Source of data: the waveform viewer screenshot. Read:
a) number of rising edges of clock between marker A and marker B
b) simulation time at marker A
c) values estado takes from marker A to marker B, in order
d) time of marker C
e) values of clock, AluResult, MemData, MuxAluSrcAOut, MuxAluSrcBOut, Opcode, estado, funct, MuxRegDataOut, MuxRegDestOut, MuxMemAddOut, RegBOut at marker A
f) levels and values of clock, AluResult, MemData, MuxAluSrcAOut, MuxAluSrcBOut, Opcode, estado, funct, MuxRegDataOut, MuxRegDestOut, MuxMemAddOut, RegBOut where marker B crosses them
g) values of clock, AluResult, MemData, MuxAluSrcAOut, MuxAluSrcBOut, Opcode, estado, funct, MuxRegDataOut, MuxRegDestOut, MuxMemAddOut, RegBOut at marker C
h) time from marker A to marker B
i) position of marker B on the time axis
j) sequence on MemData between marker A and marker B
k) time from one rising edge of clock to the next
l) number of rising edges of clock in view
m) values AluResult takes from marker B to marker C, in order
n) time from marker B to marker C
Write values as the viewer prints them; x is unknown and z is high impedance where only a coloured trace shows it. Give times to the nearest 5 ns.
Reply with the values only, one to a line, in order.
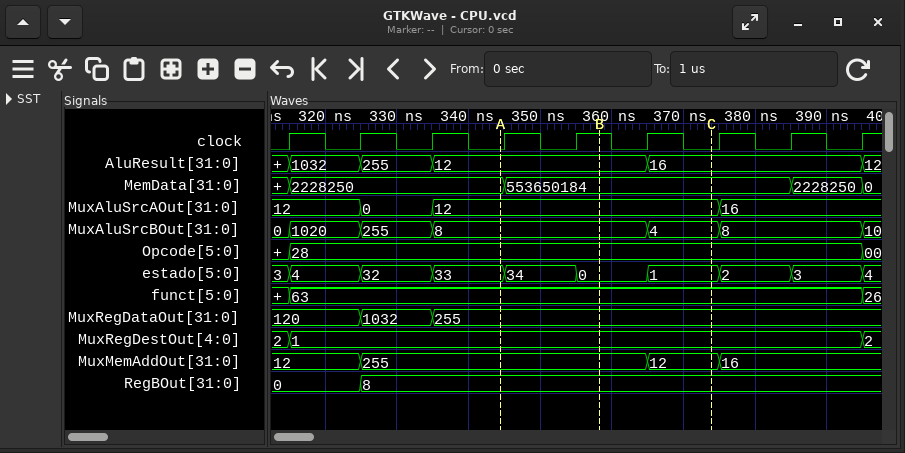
2
345 ns
33, 34, 0
375 ns
clock=0, AluResult=12, MemData=2228250, MuxAluSrcAOut=12, MuxAluSrcBOut=8, Opcode=28, estado=33, funct=63, MuxRegDataOut=255, MuxRegDestOut=1, MuxMemAddOut=255, RegBOut=8
clock=1, AluResult=12, MemData=553650184, MuxAluSrcAOut=12, MuxAluSrcBOut=8, Opcode=28, estado=0, funct=63, MuxRegDataOut=255, MuxRegDestOut=1, MuxMemAddOut=255, RegBOut=8
clock=0, AluResult=16, MemData=553650184, MuxAluSrcAOut=12, MuxAluSrcBOut=4, Opcode=28, estado=1, funct=63, MuxRegDataOut=255, MuxRegDestOut=1, MuxMemAddOut=12, RegBOut=8
15 ns
360 ns
2228250, 553650184
10 ns
9
12, 16
15 ns
